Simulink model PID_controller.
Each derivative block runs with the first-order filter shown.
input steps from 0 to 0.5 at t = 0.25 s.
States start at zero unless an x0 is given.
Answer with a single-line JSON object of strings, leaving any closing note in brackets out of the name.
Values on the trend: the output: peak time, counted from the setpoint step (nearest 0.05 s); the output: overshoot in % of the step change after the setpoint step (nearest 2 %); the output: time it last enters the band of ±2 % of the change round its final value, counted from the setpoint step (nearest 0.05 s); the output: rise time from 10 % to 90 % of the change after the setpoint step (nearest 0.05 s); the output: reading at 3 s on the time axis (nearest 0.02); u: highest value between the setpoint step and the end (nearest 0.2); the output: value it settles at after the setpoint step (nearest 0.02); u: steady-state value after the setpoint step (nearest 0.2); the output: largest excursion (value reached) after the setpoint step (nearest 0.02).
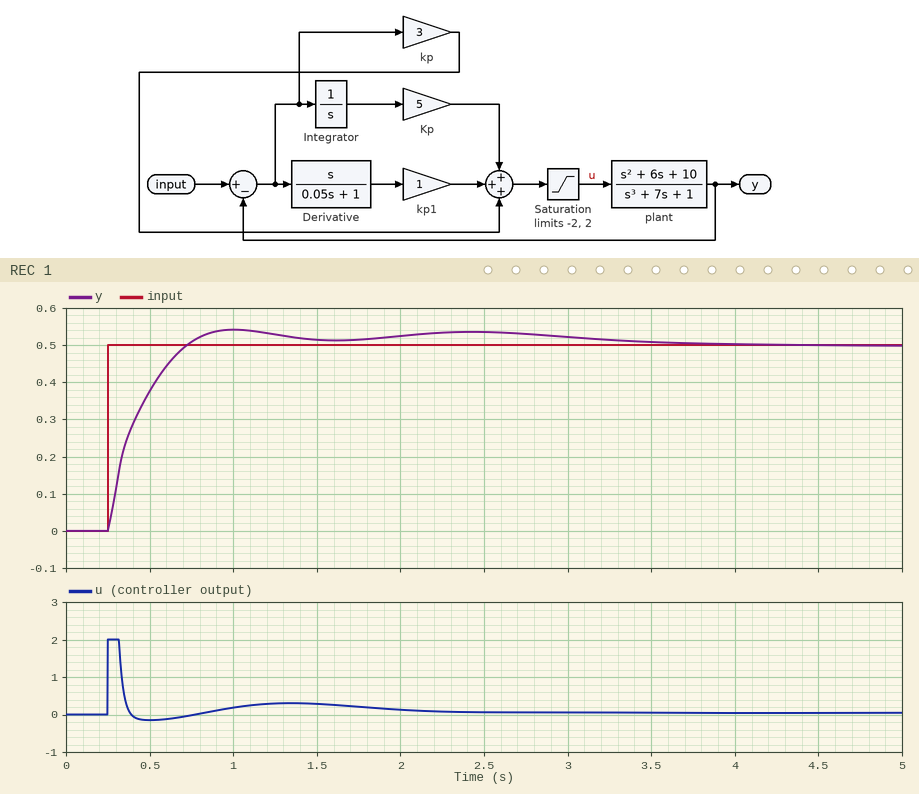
{"the output: peak time, counted from the setpoint step": "0.75 s", "the output: overshoot in % of the step change after the setpoint step": "8 %", "the output: time it last enters the band of ±2 % of the change round its final value, counted from the setpoint step": "3.15 s", "the output: rise time from 10 % to 90 % of the change after the setpoint step": "0.35 s", "the output: reading at 3 s on the time axis": "0.52", "u: highest value between the setpoint step and the end": "2.0", "the output: value it settles at after the setpoint step": "0.50", "u: steady-state value after the setpoint step": "0.0", "the output: largest excursion (value reached) after the setpoint step": "0.54"}
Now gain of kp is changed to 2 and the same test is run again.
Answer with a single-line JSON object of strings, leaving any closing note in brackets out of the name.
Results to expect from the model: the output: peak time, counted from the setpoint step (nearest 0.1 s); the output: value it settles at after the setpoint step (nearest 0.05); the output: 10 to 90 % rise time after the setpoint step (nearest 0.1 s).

{"the output: peak time, counted from the setpoint step": "0.9 s", "the output: value it settles at after the setpoint step": "0.50", "the output: 10 to 90 % rise time after the setpoint step": "0.4 s"}
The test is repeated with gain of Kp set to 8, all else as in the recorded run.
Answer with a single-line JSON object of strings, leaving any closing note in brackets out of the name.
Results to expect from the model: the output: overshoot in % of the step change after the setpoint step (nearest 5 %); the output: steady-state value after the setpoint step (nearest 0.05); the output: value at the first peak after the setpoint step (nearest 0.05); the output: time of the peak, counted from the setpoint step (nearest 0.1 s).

{"the output: overshoot in % of the step change after the setpoint step": "15 %", "the output: steady-state value after the setpoint step": "0.50", "the output: value at the first peak after the setpoint step": "0.60", "the output: time of the peak, counted from the setpoint step": "0.7 s"}
